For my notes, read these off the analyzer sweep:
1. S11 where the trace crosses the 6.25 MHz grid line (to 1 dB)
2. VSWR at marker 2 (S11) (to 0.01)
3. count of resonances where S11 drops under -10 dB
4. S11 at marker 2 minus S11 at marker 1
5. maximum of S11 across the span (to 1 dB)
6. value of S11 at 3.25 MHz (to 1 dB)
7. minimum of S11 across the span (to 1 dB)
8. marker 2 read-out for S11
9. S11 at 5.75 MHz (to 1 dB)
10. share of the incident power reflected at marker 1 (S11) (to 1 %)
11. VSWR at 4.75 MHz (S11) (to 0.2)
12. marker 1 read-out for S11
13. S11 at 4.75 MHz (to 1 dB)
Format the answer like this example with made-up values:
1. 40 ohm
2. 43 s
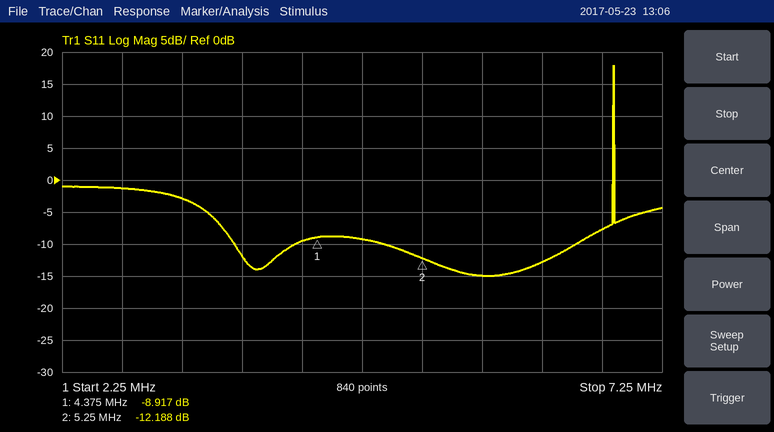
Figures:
1. -13 dB
2. 1.65
3. 2
4. -3.271 dB
5. 18 dB
6. -3 dB
7. -15 dB
8. -12.188 dB
9. -15 dB
10. 13 %
11. 2.0
12. -8.917 dB
13. -9 dB
